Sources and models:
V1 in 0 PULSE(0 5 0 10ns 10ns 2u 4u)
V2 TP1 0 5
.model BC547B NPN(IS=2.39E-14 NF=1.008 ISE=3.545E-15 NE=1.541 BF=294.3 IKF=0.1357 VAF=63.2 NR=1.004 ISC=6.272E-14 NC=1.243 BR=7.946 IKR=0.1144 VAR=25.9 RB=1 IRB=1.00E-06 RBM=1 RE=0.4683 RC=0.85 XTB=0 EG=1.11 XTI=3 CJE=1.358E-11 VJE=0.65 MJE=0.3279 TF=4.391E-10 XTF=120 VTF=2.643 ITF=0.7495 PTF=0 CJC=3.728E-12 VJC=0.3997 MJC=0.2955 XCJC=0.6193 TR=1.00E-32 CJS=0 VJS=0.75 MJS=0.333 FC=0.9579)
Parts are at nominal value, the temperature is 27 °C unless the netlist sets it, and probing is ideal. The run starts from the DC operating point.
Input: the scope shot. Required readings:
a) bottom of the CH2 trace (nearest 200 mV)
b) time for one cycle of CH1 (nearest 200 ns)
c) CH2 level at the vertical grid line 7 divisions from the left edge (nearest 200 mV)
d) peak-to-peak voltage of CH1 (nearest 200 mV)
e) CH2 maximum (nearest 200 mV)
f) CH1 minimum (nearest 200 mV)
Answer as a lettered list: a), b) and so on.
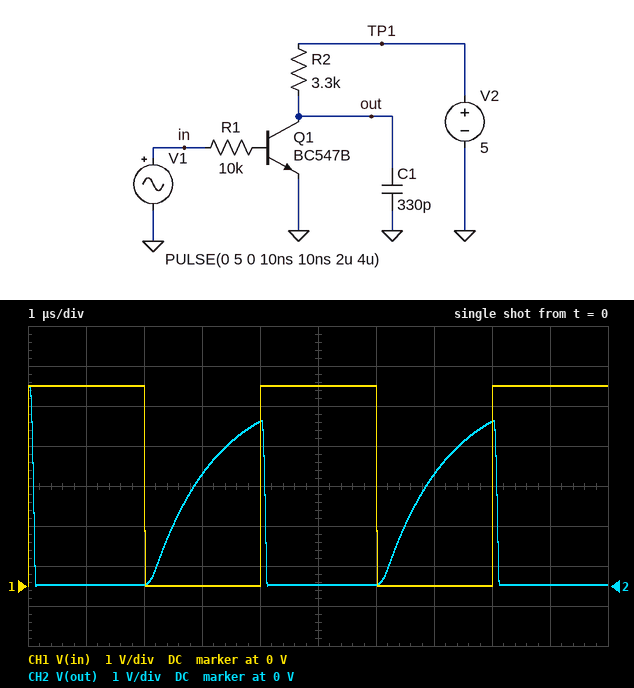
a) 0 V
b) 4.0 µs
c) 2.8 V
d) 5.0 V
e) 5.0 V
f) 0 V
